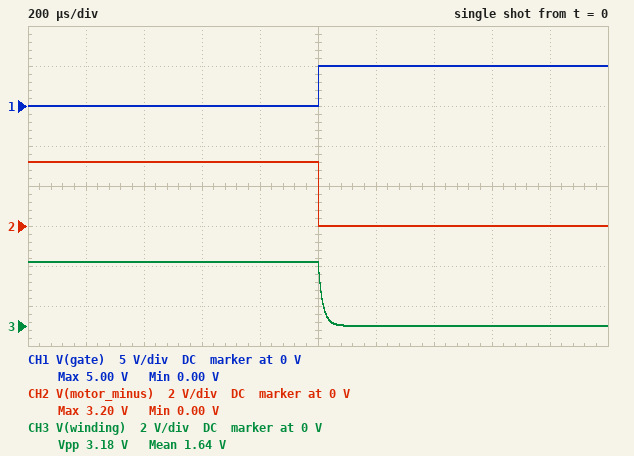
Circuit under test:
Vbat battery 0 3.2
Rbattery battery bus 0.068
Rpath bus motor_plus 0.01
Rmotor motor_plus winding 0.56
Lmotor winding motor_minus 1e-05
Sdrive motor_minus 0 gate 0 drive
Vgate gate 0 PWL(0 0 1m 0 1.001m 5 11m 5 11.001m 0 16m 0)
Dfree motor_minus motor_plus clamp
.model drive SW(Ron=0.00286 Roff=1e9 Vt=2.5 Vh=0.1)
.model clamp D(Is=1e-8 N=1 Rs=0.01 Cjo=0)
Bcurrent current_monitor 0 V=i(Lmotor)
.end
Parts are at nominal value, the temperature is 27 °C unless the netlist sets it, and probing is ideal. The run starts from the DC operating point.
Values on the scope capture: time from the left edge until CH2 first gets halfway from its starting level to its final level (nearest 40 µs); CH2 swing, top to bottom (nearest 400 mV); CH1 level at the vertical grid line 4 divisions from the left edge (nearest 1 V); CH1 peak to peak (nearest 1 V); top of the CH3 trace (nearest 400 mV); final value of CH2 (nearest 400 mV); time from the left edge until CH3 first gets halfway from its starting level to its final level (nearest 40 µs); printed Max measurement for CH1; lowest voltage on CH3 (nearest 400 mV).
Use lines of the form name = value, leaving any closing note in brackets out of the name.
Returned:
time from the left edge until CH2 first gets halfway from its starting level to its final level = 1.00 ms
CH2 swing, top to bottom = 3.2 V
CH1 level at the vertical grid line 4 divisions from the left edge = 0 V
CH1 peak to peak = 5 V
top of the CH3 trace = 3.2 V
final value of CH2 = 0 V
time from the left edge until CH3 first gets halfway from its starting level to its final level = 1.00 ms
printed Max measurement for CH1 = 5.00 V
lowest voltage on CH3 = 0 V
